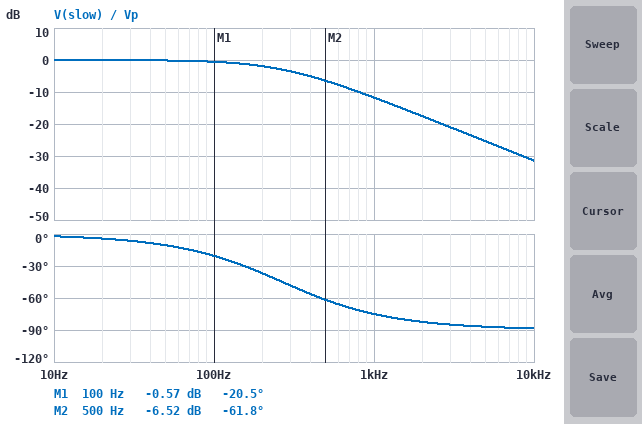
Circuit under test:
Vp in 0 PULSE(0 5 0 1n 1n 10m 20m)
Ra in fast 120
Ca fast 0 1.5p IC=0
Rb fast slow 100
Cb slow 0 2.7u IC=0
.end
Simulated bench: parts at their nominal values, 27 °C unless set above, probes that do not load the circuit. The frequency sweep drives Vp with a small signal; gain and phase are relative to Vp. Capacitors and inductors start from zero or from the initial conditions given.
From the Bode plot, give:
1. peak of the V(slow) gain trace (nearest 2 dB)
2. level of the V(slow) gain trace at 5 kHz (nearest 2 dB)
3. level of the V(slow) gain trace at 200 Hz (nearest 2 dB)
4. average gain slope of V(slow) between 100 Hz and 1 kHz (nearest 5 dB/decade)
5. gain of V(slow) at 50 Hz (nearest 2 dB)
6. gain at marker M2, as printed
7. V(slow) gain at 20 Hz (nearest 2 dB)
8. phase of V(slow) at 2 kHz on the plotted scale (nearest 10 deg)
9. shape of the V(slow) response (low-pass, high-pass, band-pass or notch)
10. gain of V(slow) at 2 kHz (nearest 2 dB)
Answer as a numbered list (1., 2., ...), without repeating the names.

1. 0 dB
2. -26 dB
3. -2 dB
4. -10 dB/decade
5. 0 dB
6. -6.52 dB
7. 0 dB
8. -80 deg
9. low-pass
10. -18 dB
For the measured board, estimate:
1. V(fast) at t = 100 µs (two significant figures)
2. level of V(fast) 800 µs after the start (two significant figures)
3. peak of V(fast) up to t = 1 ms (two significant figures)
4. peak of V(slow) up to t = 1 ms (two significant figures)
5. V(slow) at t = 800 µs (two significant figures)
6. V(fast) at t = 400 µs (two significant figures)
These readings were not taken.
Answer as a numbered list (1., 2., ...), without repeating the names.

1. 2.7 V
2. 4.3 V
3. 4.5 V
4. 4.1 V
5. 3.7 V
6. 3.6 V
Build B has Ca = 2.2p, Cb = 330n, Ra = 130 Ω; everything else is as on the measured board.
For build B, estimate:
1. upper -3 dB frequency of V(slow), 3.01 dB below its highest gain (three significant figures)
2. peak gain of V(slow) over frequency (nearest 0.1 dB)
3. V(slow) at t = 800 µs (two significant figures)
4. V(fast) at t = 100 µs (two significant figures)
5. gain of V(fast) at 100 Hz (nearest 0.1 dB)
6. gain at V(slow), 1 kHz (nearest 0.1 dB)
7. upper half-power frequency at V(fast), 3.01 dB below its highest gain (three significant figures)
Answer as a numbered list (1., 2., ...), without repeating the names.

1. 2.10 kHz
2. 0 dB
3. 5.0 V
4. 4.2 V
5. 0 dB
6. -0.9 dB
7. 2.66 kHz
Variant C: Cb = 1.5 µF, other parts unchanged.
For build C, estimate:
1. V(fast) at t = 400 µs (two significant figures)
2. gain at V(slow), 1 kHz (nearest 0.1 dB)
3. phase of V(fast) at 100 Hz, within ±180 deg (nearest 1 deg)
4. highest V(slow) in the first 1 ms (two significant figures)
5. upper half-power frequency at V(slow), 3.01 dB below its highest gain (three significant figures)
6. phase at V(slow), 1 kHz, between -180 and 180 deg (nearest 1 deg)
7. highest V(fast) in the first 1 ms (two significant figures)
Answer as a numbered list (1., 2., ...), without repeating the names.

1. 4.2 V
2. -7.2 dB
3. -6 deg
4. 4.8 V
5. 482 Hz
6. -64 deg
7. 4.9 V
